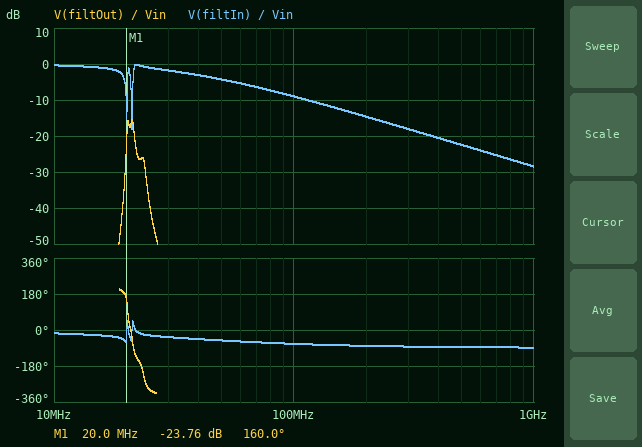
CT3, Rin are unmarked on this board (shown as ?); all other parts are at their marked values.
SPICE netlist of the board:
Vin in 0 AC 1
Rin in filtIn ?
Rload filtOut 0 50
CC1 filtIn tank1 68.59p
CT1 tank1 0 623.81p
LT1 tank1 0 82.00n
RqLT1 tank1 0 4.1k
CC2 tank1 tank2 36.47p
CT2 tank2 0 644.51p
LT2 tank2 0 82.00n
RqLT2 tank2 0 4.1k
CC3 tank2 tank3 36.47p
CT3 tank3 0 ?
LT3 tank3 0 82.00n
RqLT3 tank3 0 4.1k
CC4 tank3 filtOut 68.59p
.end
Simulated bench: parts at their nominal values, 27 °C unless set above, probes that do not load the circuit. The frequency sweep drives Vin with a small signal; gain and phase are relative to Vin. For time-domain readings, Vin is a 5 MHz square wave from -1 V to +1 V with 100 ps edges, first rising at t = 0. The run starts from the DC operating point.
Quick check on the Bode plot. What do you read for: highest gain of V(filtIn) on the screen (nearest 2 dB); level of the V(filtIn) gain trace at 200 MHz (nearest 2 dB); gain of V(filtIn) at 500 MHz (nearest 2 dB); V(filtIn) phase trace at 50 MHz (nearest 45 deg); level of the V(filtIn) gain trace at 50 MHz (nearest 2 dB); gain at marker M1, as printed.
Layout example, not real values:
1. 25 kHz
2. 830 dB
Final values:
1. 0 dB
2. -14 dB
3. -22 dB
4. -45 deg
5. -4 dB
6. -23.76 dB
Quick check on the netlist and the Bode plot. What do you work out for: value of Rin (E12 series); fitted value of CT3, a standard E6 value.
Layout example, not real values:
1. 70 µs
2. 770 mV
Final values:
1. 68 Ω
2. 470 pF
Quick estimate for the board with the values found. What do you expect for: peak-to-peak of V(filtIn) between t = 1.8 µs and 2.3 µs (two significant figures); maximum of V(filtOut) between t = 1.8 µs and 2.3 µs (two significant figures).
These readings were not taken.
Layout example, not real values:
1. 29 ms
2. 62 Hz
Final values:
1. 2.1 V
2. 3.1 mV
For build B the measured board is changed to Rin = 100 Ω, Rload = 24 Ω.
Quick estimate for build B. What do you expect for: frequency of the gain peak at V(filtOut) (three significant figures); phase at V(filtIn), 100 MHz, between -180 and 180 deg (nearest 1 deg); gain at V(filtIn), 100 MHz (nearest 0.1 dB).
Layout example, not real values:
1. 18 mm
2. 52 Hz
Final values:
1. 20.4 MHz
2. -76 deg
3. -12.1 dB
